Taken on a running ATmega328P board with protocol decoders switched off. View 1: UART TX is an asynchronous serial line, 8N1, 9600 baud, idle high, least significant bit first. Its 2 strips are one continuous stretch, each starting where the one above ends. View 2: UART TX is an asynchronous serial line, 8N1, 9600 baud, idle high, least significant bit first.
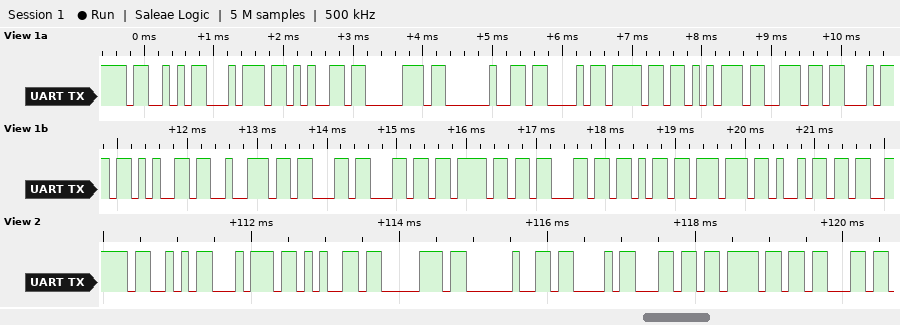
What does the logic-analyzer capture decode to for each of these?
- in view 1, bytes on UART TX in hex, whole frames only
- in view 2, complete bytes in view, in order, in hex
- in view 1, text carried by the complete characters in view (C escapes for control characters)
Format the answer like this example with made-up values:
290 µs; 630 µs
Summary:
0x53 0x74 0x65 0x70 0x20 0x43 0x6F 0x75 0x6E 0x74 0x65 0x72 0x63 0x6C 0x6F 0x63 0x6B 0x77 0x69; 53 74 65 70 20 43 6C 6F 63; "Step Counterclockwi"
